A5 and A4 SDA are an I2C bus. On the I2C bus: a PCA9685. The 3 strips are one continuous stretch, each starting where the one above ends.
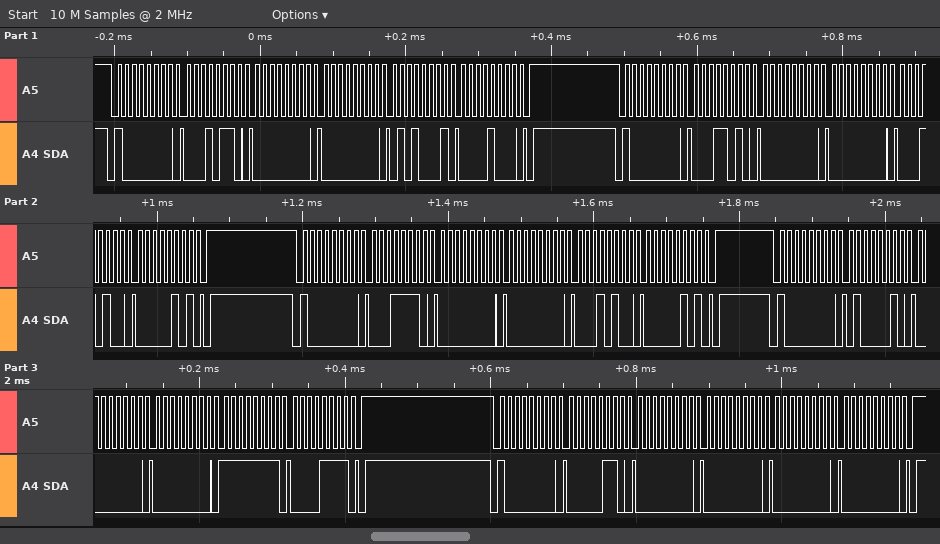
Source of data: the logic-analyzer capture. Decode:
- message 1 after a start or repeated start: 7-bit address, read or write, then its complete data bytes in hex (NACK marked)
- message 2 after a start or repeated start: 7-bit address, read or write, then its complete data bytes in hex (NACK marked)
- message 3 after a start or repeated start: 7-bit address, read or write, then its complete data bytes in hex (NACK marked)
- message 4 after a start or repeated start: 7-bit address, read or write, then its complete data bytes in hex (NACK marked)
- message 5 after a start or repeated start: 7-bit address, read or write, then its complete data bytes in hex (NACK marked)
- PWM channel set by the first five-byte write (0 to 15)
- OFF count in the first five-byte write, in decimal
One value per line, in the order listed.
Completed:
0x40 write: 16 00 00 51 08
0x40 write: 1A 00 00 14 05
0x40 write: 1E 00 00 14 05
0x40 write: 42 00 00 FF 0F
0x40 write: 06 00 00 00 00
4
2129
